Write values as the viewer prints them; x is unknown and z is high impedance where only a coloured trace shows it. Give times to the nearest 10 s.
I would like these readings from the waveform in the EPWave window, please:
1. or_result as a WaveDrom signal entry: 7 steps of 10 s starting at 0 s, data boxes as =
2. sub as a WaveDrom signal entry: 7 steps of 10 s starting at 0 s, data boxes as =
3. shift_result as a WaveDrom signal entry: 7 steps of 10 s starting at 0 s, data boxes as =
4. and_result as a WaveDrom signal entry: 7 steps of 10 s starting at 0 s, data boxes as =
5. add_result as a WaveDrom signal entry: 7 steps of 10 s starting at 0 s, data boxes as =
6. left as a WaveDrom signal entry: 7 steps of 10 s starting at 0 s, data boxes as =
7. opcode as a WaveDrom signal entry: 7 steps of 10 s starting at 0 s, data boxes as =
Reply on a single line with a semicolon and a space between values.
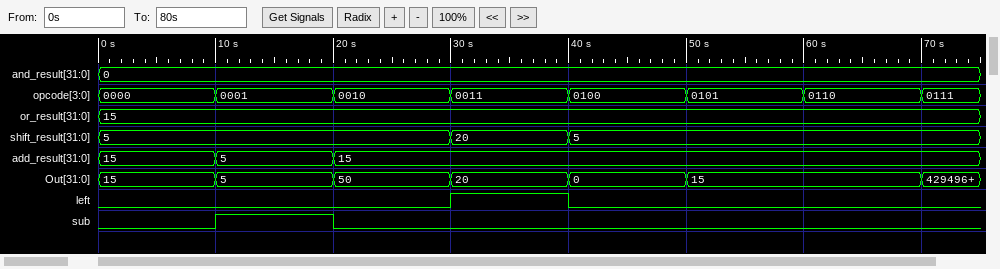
{name: 'or_result', wave: '=......', data: '15'}; {name: 'sub', wave: '010....'}; {name: 'shift_result', wave: '=..==..', data: '5 20 5'}; {name: 'and_result', wave: '=......', data: '0'}; {name: 'add_result', wave: '===....', data: '15 5 15'}; {name: 'left', wave: '0..10..'}; {name: 'opcode', wave: '=======', data: '0000 0001 0010 0011 0100 0101 0110'}
